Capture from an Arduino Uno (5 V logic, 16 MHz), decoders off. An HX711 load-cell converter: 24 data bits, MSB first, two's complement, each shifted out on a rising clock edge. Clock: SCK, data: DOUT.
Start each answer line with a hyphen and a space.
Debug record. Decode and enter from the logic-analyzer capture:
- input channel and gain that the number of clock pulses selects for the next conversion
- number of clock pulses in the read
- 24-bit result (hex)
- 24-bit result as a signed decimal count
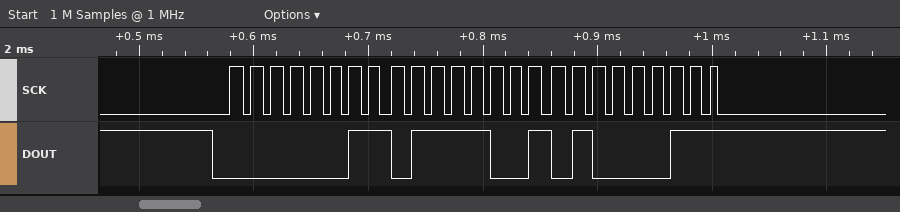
- channel A, gain 128
- 25
- 0x037943
- 227651
